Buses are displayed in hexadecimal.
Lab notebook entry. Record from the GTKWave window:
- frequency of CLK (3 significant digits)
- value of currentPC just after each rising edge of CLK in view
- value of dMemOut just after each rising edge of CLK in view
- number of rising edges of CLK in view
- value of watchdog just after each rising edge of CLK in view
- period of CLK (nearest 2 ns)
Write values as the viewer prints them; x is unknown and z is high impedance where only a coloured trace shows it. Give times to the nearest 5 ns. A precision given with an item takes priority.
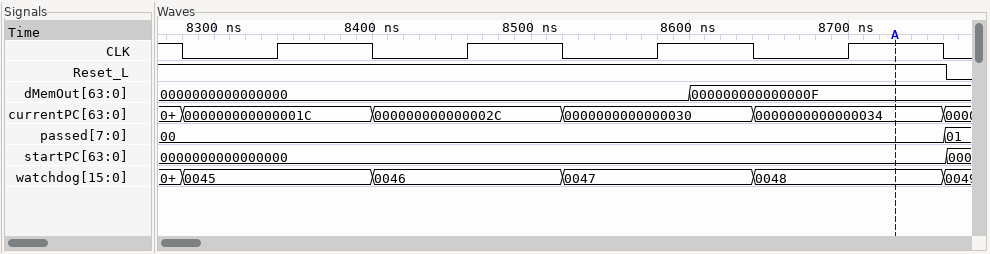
8.33 MHz
000000000000001C, 000000000000002C, 0000000000000030, 0000000000000034
0000000000000000, 0000000000000000, 0000000000000000, 000000000000000F
4
0045, 0046, 0047, 0048
120 ns
